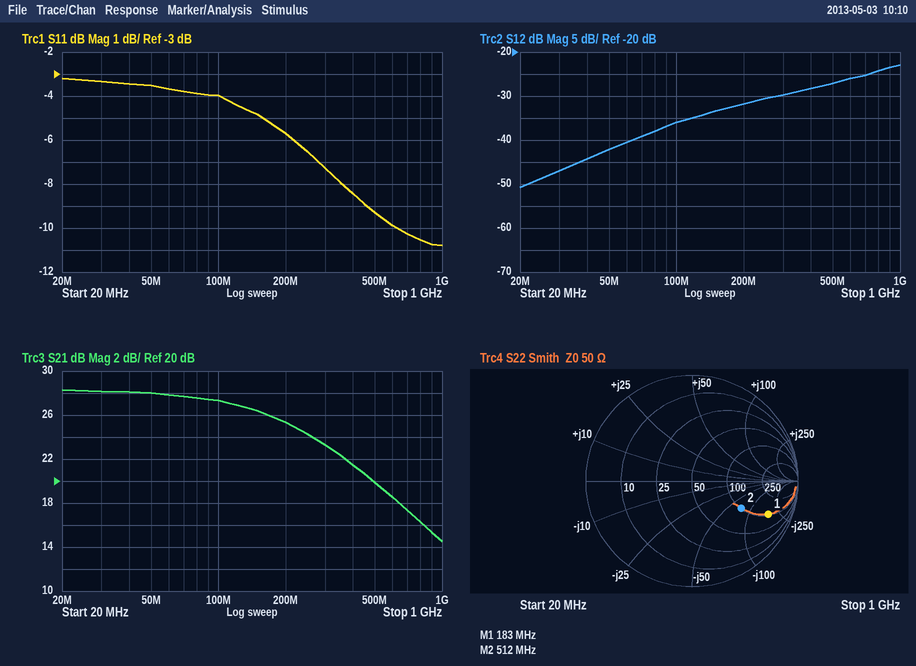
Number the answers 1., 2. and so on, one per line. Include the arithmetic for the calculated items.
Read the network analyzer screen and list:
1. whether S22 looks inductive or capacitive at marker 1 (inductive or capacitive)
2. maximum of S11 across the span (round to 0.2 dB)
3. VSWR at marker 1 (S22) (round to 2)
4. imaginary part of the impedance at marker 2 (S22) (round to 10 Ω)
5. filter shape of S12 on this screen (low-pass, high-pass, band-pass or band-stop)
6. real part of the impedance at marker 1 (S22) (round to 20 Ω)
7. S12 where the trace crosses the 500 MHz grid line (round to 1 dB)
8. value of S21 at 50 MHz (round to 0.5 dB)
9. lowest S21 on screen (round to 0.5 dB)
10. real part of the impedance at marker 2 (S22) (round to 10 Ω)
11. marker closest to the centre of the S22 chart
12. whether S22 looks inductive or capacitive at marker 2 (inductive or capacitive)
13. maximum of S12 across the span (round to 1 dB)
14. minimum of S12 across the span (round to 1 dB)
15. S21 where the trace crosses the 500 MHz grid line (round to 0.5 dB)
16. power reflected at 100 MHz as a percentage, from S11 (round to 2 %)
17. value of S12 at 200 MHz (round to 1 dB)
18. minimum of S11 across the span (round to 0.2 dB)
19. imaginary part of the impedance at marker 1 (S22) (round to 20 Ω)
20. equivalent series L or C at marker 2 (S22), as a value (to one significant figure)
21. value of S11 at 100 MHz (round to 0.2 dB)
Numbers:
1. capacitive
2. -3.2 dB
3. 8
4. -70 Ω
5. high-pass
6. 100 Ω
7. -27 dB
8. 28.0 dB
9. 14.5 dB
10. 100 Ω
11. marker 2
12. capacitive
13. -23 dB
14. -51 dB
15. 20.0 dB
16. 10^(-4/10) ≈ 40 %
17. -32 dB
18. -10.8 dB
19. -180 Ω
20. C = 1/(2π × 512 MHz × 70 Ω) ≈ 4 pF
21. -4.0 dB
